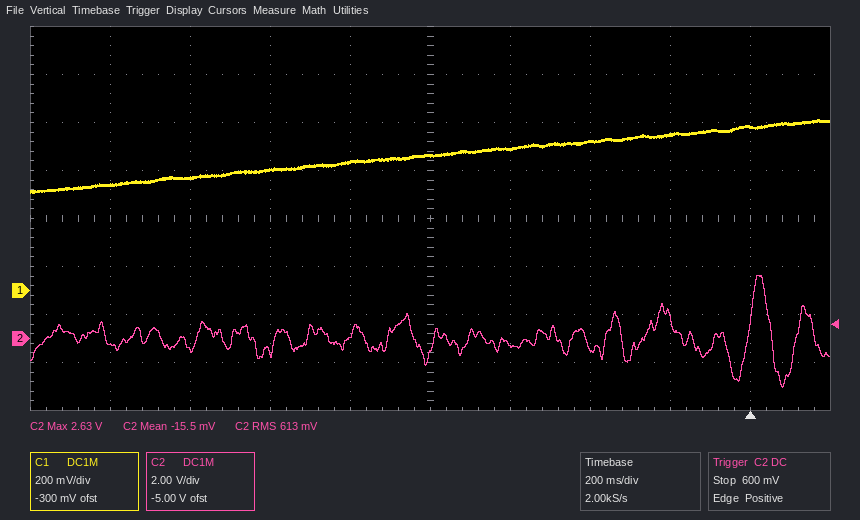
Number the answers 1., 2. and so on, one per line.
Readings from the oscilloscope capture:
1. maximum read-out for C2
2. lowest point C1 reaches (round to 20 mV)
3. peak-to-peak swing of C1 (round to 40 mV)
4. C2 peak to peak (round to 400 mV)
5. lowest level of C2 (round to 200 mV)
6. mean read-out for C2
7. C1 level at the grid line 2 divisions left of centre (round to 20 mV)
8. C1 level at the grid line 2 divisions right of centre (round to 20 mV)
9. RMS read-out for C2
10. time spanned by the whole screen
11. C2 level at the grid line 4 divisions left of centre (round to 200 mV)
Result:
1. 2.63 V
2. 400 mV
3. 320 mV
4. 4.8 V
5. -2.0 V
6. -15.5 mV
7. 500 mV
8. 620 mV
9. 613 mV
10. 2 s
11. -200 mV
